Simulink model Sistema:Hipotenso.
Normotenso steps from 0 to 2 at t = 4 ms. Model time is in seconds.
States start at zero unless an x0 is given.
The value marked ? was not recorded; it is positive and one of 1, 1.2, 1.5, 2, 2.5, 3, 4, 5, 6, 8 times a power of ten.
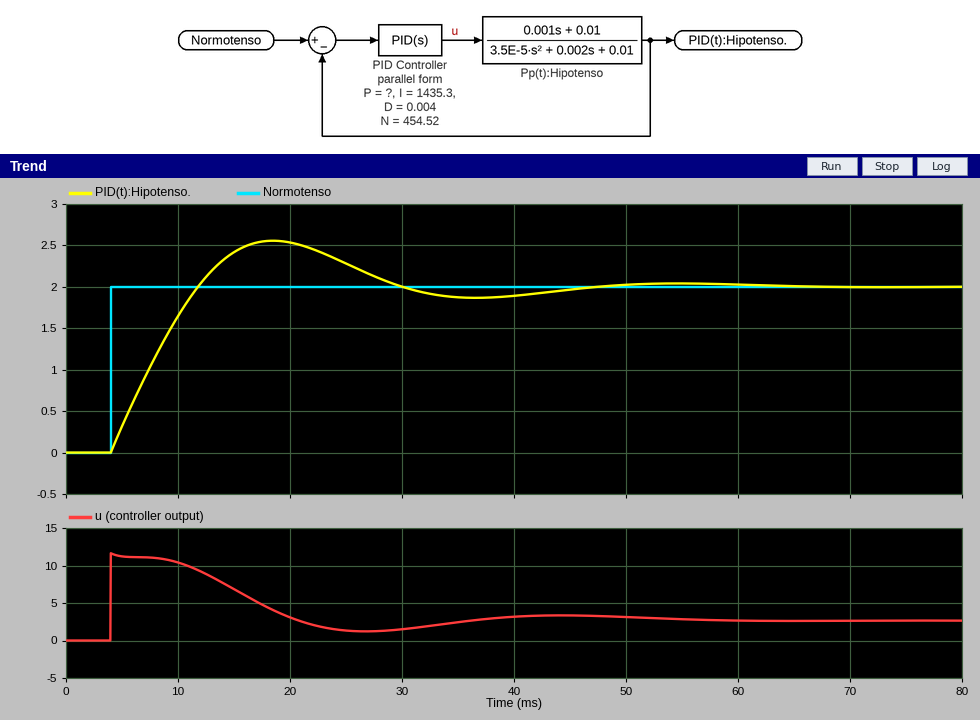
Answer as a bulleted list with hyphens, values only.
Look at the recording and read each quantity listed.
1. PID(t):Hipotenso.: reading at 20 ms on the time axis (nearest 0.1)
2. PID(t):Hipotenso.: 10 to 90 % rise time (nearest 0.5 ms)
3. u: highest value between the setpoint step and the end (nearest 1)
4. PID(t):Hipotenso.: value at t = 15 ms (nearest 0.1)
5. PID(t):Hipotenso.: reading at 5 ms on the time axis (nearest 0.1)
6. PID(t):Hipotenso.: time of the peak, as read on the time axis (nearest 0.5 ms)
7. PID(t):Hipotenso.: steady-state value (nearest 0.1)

- 2.5
- 6.0 ms
- 12
- 2.4
- 0.3
- 18.5 ms
- 2.0
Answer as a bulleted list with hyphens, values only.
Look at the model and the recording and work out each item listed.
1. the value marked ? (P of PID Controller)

- 4
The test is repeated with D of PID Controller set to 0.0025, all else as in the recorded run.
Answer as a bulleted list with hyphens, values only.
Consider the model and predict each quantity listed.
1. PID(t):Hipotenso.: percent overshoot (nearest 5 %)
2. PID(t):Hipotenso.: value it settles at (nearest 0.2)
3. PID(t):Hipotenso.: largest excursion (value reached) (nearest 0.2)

- 30 %
- 2.0
- 2.6
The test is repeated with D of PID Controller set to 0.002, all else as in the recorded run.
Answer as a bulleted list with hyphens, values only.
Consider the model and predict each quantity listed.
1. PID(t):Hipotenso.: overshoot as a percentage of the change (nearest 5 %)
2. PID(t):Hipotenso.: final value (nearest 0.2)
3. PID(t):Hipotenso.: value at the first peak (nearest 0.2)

- 30 %
- 2.0
- 2.6
